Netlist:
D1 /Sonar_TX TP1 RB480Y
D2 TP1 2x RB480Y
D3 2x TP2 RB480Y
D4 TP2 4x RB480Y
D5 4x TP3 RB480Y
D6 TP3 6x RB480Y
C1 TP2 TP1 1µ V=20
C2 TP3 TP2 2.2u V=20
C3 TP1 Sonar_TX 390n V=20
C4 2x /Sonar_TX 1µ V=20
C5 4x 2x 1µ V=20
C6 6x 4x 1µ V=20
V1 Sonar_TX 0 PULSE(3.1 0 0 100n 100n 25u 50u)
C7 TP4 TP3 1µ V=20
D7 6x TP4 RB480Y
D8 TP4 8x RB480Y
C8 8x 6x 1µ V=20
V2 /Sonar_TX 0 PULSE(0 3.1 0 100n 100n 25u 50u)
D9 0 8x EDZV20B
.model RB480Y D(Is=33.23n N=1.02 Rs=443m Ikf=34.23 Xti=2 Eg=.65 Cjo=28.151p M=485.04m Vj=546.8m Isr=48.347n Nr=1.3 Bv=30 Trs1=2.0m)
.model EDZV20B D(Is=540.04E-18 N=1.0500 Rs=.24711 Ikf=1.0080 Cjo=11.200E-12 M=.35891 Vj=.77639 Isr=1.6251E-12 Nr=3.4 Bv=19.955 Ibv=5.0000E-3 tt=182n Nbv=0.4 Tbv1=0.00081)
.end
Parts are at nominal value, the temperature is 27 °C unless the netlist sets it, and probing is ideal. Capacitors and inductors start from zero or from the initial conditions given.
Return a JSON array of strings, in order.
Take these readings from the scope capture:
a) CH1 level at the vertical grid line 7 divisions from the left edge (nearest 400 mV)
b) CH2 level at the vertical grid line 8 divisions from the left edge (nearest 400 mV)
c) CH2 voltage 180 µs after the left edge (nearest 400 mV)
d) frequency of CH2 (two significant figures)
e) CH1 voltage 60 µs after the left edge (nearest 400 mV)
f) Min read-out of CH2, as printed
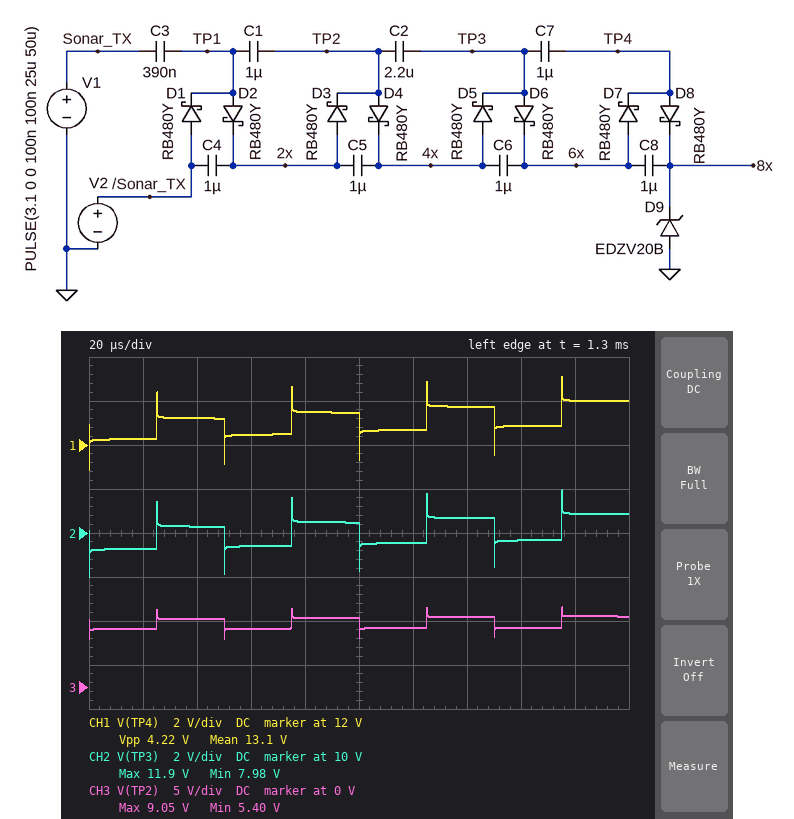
["13.6 V", "9.6 V", "10.8 V", "20 kHz", "12.4 V", "7.98 V"]
